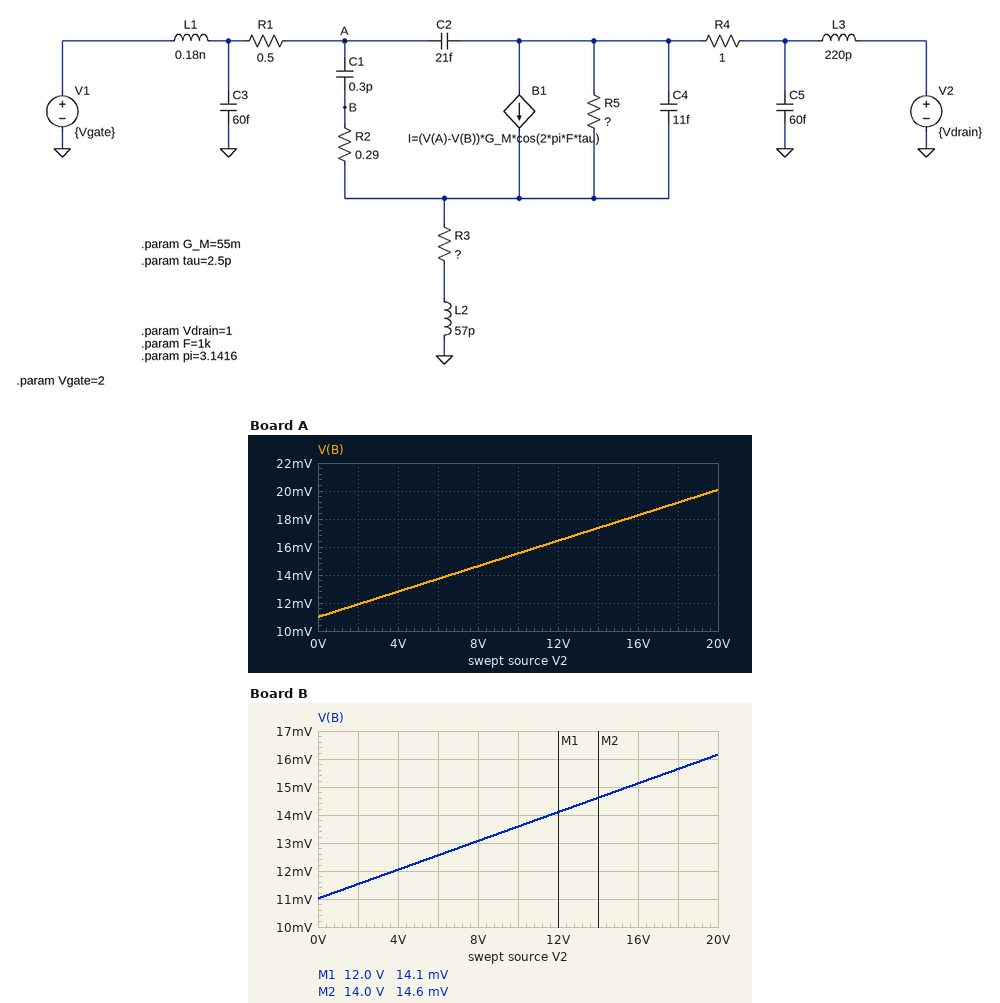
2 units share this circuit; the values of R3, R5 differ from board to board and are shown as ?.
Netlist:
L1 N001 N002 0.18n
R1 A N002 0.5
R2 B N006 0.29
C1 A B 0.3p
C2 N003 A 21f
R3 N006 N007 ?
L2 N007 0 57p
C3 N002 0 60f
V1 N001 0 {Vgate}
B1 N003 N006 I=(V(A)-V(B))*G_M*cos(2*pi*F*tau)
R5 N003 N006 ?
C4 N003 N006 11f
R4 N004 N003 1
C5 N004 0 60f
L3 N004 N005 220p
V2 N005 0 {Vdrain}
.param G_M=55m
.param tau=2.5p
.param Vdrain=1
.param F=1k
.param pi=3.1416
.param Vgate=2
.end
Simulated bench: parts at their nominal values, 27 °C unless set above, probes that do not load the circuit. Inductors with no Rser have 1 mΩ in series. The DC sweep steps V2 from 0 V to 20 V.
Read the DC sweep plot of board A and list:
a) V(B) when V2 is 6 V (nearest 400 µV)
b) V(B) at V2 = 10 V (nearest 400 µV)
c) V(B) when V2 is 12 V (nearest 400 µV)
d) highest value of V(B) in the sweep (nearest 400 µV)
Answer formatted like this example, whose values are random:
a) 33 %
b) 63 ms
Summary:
a) 13.6 mV
b) 15.6 mV
c) 16.4 mV
d) 20.0 mV
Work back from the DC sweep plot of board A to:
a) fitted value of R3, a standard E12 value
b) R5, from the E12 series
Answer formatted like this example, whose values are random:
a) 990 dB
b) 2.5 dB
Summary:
a) 0.1 Ω
b) 220 Ω
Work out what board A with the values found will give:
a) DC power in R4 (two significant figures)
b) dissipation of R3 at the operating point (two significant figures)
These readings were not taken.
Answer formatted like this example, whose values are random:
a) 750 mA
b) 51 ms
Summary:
a) 13 mW
b) 1.3 mW
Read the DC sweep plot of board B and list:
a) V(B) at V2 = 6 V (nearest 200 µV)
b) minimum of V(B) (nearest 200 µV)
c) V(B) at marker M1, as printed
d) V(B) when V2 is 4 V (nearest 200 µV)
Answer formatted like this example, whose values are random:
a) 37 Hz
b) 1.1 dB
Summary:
a) 12.6 mV
b) 11.0 mV
c) 14.1 mV
d) 12.0 mV
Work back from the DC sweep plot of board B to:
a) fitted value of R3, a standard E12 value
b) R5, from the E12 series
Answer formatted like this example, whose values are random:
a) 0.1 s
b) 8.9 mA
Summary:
a) 0.1 Ω
b) 390 Ω
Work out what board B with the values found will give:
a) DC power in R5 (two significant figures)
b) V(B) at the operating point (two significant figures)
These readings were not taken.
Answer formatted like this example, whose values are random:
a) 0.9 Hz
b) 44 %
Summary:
a) 2.0 mW
b) 11 mV
